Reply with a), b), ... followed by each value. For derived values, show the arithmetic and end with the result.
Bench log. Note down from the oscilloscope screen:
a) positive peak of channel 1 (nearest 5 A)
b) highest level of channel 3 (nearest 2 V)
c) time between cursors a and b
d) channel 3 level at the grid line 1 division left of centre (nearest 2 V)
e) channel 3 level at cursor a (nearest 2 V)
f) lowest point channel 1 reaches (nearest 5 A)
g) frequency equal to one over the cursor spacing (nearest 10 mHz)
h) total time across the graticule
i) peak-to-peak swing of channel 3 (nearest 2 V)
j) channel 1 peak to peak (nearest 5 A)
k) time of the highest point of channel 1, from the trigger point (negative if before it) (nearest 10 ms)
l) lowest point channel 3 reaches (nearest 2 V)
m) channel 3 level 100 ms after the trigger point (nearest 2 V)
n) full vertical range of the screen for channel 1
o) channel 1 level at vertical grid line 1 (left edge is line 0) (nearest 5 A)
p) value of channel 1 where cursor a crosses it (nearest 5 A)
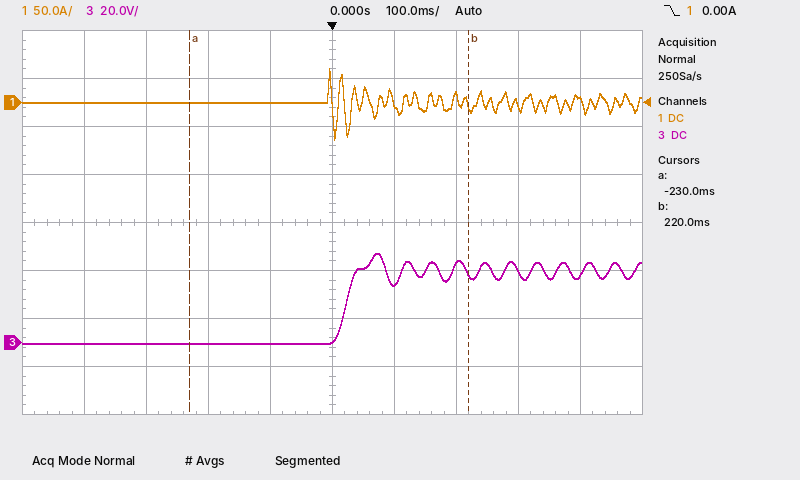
a) 35 A
b) 38 V
c) 220 ms − (-230 ms) = 450 ms
d) 0 V
e) 0 V
f) -40 A
g) 1 / 450 ms ≈ 2.22 Hz
h) 1 s
i) 38 V − (0 V) = 38 V
j) 35 A − (-40 A) = 75 A
k) 0 ms
l) 0 V
m) 24 V
n) 400 A
o) 0 A
p) 0 A
